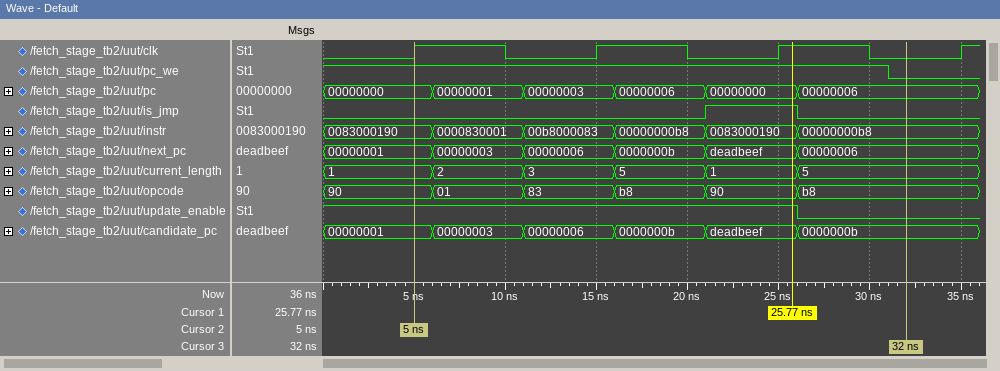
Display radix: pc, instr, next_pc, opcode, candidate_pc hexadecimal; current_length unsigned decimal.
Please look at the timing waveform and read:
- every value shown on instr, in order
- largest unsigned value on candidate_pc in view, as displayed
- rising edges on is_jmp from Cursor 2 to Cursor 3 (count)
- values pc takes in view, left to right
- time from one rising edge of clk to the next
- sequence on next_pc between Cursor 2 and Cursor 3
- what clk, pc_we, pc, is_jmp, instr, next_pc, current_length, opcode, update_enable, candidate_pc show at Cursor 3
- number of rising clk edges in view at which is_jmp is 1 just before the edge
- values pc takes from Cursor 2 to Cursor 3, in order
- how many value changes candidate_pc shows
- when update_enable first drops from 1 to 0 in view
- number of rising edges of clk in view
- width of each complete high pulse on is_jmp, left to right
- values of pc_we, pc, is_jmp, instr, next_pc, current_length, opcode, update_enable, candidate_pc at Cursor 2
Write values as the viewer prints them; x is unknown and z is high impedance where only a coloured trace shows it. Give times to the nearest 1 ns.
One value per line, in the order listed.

0083000190, 0000830001, 00b8000083, 00000000b8, 0083000190, 00000000b8
deadbeef
1
00000000, 00000001, 00000003, 00000006, 00000000, 00000006
10 ns
00000001, 00000003, 00000006, 0000000b, deadbeef, 00000006
clk=0, pc_we=0, pc=00000006, is_jmp=0, instr=00000000b8, next_pc=00000006, current_length=5, opcode=b8, update_enable=0, candidate_pc=0000000b
1
00000000, 00000001, 00000003, 00000006, 00000000, 00000006
5
26 ns
4
5 ns
pc_we=1, pc=00000000, is_jmp=0, instr=0083000190, next_pc=00000001, current_length=1, opcode=90, update_enable=1, candidate_pc=00000001
